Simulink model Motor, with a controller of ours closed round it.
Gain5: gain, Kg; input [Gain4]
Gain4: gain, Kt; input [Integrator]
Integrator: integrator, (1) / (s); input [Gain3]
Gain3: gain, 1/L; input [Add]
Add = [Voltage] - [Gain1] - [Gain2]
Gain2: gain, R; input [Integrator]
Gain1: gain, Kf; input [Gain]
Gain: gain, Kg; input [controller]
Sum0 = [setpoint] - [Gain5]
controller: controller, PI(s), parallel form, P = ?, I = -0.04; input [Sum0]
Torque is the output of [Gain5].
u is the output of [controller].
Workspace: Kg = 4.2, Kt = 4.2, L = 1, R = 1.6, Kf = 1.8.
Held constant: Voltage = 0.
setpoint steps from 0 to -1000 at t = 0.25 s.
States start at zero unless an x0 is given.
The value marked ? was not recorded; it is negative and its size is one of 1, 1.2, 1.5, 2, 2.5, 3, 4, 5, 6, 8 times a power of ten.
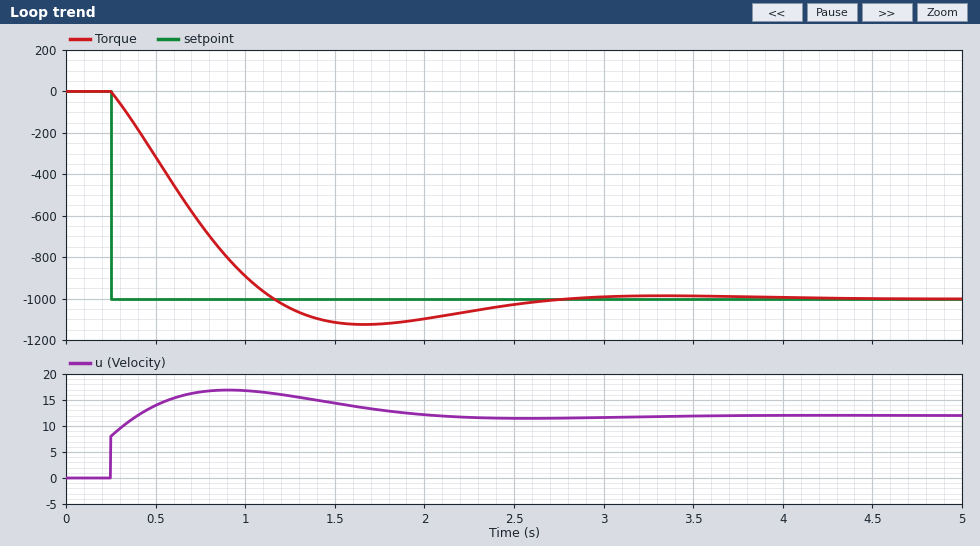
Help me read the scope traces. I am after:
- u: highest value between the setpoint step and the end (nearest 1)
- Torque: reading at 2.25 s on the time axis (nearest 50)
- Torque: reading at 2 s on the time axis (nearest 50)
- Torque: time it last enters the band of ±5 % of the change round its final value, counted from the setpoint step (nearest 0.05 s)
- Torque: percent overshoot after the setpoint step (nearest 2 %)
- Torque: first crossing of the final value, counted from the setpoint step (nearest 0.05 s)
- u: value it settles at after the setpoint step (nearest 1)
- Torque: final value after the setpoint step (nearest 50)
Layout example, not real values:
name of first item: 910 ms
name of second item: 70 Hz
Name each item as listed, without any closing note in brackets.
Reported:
u: highest value between the setpoint step and the end: 17
Torque: reading at 2.25 s on the time axis: -1050
Torque: reading at 2 s on the time axis: -1100
Torque: time it last enters the band of ±5 % of the change round its final value, counted from the setpoint step: 2.10 s
Torque: percent overshoot after the setpoint step: 12 %
Torque: first crossing of the final value, counted from the setpoint step: 0.90 s
u: value it settles at after the setpoint step: 12
Torque: final value after the setpoint step: -1000
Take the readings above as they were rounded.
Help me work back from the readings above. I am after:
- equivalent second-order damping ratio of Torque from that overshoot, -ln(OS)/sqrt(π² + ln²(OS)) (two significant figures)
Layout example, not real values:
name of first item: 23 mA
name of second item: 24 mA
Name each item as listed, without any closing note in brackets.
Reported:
equivalent second-order damping ratio of Torque from that overshoot, -ln(OS)/sqrt(π² + ln²(OS)): 0.56
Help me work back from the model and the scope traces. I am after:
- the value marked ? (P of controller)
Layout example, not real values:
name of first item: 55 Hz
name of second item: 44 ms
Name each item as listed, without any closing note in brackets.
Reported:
the value marked ?: -0.008
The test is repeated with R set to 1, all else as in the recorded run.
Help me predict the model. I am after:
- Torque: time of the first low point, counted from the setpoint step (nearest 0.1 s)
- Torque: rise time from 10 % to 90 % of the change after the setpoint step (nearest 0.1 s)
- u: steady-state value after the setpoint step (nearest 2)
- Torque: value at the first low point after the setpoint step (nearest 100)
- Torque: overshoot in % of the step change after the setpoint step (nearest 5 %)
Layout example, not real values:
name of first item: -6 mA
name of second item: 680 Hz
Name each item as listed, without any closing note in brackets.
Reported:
Torque: time of the first low point, counted from the setpoint step: 1.3 s
Torque: rise time from 10 % to 90 % of the change after the setpoint step: 0.6 s
u: steady-state value after the setpoint step: 8
Torque: value at the first low point after the setpoint step: -1200
Torque: overshoot in % of the step change after the setpoint step: 25 %
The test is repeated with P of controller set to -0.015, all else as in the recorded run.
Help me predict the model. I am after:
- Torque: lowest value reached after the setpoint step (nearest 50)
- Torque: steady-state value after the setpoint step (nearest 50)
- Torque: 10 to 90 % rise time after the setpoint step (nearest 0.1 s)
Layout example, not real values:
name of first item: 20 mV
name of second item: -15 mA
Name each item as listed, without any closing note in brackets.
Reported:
Torque: lowest value reached after the setpoint step: -1050
Torque: steady-state value after the setpoint step: -1000
Torque: 10 to 90 % rise time after the setpoint step: 0.7 s
